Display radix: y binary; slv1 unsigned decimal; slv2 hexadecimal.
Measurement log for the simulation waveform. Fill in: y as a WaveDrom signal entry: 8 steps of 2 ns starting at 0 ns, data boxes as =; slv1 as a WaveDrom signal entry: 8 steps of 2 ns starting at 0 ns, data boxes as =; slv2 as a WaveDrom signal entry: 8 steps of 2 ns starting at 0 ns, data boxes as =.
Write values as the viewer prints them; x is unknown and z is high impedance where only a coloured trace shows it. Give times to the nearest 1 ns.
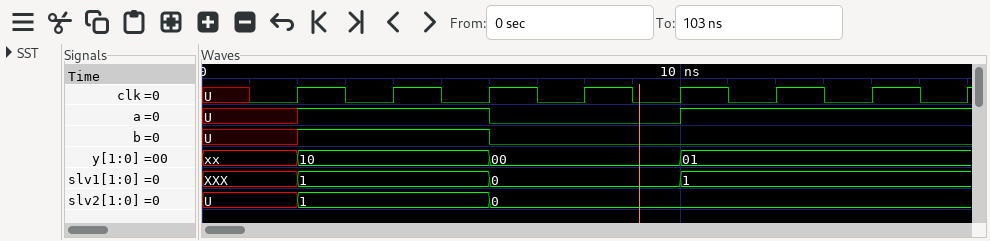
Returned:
{name: 'y', wave: 'x=.=.=..', data: '10 00 01'}
{name: 'slv1', wave: '==.=.=..', data: 'XXX 1 0 1'}
{name: 'slv2', wave: '==.=....', data: 'U 1 0'}
